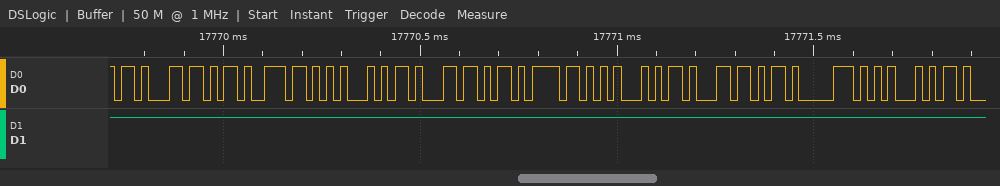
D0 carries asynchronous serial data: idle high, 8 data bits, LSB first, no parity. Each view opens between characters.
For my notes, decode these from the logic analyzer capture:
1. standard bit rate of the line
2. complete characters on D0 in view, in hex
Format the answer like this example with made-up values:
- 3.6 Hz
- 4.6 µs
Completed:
- 57600 baud
- 8B, 6B, 6E, 45, 8B, 6B, 6F, 45, 8B, 6B, 70, 45
